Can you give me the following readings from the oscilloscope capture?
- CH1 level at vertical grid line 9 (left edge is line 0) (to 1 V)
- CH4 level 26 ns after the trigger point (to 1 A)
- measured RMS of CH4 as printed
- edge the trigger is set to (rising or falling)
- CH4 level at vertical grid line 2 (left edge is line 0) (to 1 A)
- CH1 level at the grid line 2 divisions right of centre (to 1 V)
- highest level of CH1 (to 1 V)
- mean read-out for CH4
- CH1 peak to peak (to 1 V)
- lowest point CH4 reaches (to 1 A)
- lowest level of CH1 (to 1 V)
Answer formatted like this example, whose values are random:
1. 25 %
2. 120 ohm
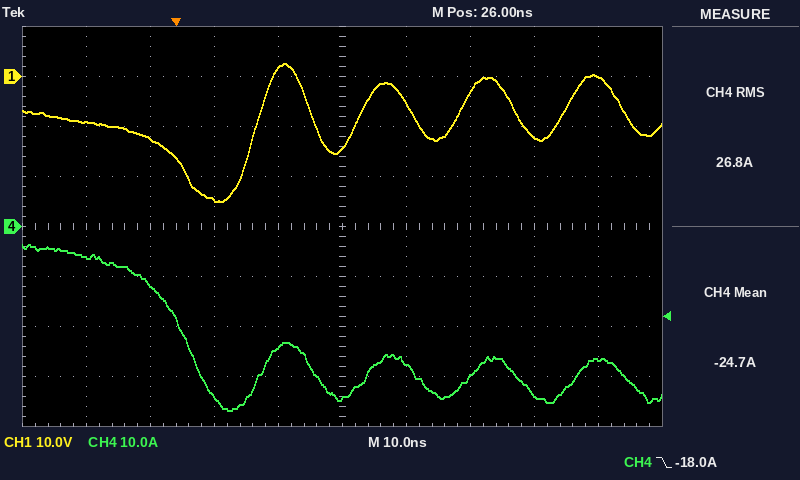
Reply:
1. 0 V
2. -34 A
3. 26.8 A
4. falling
5. -12 A
6. -3 V
7. 3 V
8. -24.7 A
9. 28 V
10. -37 A
11. -25 V
